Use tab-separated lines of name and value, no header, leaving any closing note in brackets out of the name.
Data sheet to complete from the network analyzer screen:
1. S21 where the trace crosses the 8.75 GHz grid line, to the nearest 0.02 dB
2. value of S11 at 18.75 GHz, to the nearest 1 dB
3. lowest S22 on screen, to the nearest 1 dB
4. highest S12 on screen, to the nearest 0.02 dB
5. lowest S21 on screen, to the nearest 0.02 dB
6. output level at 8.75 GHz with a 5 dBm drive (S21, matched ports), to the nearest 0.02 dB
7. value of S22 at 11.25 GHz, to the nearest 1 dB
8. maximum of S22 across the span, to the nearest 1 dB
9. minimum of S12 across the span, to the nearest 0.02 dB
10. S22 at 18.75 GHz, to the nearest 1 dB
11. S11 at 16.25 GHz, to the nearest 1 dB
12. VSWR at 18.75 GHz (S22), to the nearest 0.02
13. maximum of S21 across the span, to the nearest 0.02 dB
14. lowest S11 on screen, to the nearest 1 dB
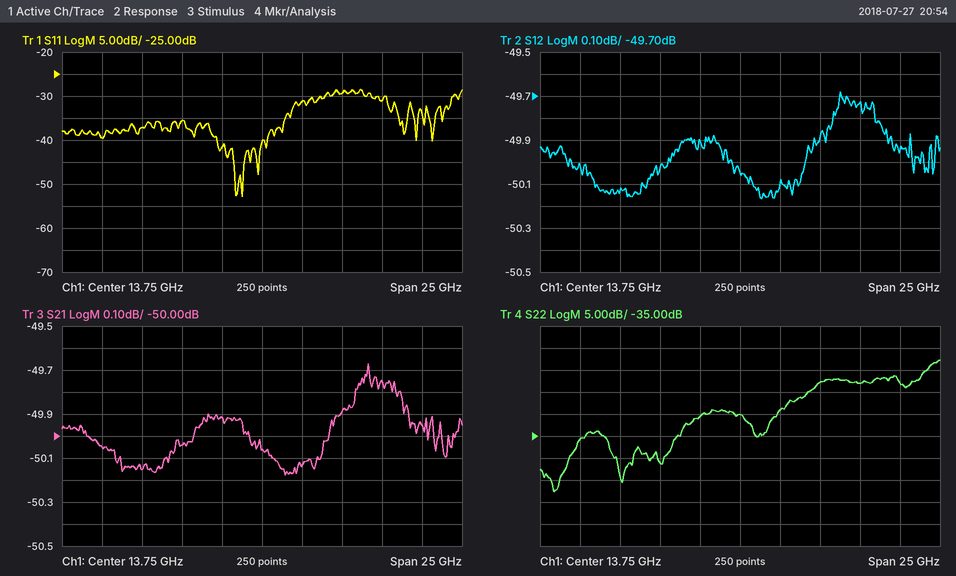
S21 where the trace crosses the 8.75 GHz grid line, to the nearest 0.02 dB	-50.04 dB
value of S11 at 18.75 GHz, to the nearest 1 dB	-29 dB
lowest S22 on screen, to the nearest 1 dB	-48 dB
highest S12 on screen, to the nearest 0.02 dB	-49.68 dB
lowest S21 on screen, to the nearest 0.02 dB	-50.18 dB
output level at 8.75 GHz with a 5 dBm drive (S21, matched ports), to the nearest 0.02 dB	-45.04 dBm
value of S22 at 11.25 GHz, to the nearest 1 dB	-31 dB
maximum of S22 across the span, to the nearest 1 dB	-18 dB
minimum of S12 across the span, to the nearest 0.02 dB	-50.16 dB
S22 at 18.75 GHz, to the nearest 1 dB	-23 dB
S11 at 16.25 GHz, to the nearest 1 dB	-31 dB
VSWR at 18.75 GHz (S22), to the nearest 0.02	1.16
maximum of S21 across the span, to the nearest 0.02 dB	-49.68 dB
lowest S11 on screen, to the nearest 1 dB	-53 dB
